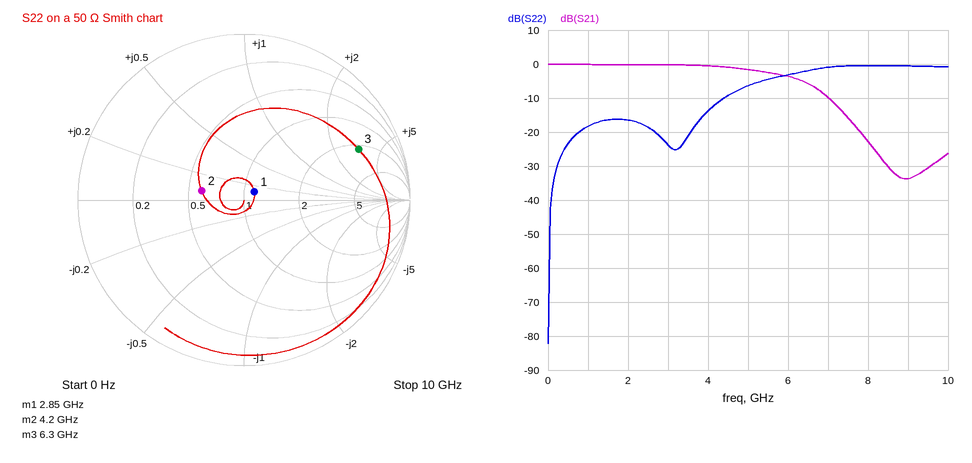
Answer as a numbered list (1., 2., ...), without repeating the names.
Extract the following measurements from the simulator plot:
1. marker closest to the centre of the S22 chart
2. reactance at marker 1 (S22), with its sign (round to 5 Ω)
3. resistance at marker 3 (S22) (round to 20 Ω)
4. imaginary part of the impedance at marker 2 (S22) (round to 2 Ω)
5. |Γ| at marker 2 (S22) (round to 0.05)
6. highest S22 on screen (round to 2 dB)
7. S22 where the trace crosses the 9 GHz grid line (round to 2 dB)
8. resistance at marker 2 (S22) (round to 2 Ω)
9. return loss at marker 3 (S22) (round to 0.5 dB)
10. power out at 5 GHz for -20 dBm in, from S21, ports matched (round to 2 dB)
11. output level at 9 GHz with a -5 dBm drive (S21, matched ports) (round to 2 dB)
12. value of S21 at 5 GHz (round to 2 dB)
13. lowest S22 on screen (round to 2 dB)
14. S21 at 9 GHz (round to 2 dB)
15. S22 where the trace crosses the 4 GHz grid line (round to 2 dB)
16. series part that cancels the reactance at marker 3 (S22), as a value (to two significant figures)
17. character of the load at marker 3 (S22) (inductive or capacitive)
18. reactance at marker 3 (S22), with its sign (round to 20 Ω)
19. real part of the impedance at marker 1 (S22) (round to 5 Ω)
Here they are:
1. marker 1
2. +5 Ω
3. 120 Ω
4. +4 Ω
5. 0.25
6. 0 dB
7. 0 dB
8. 30 Ω
9. 2.5 dB
10. -22 dBm
11. -38 dBm
12. -2 dB
13. -82 dB
14. -34 dB
15. -14 dB
16. 160 fF
17. inductive
18. +160 Ω
19. 55 Ω
